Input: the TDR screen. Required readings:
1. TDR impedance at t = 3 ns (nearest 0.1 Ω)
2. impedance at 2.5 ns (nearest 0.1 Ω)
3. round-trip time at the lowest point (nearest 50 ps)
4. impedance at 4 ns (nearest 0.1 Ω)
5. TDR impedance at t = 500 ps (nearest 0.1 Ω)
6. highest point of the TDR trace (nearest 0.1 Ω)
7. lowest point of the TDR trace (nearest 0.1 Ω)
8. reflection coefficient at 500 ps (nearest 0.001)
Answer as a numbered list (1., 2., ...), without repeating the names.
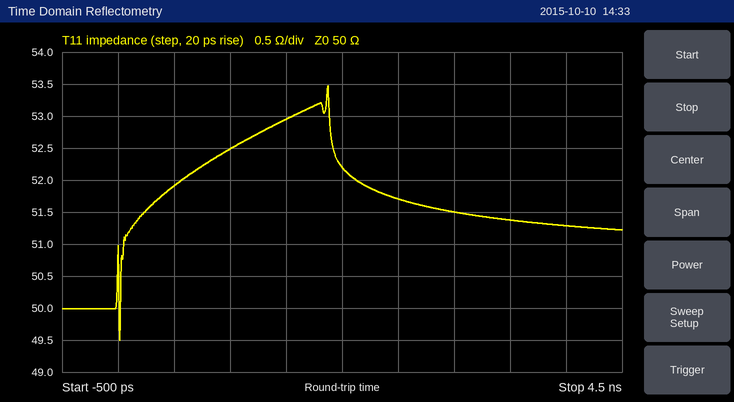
1. 51.5 Ω
2. 51.7 Ω
3. 0 ps
4. 51.3 Ω
5. 51.9 Ω
6. 53.5 Ω
7. 49.5 Ω
8. +0.019
